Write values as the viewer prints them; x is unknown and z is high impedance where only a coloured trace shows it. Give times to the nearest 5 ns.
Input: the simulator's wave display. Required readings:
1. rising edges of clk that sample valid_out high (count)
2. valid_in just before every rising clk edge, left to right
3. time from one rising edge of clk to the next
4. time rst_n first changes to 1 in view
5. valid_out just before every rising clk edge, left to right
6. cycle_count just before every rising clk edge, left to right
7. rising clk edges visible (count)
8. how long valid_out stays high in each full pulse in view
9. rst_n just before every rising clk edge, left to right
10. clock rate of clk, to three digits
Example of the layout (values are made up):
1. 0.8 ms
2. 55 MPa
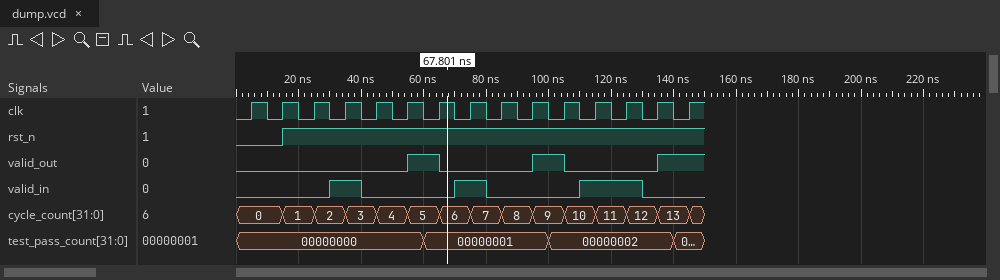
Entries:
1. 3
2. 0 0 0 1 0 0 0 1 0 0 0 1 1 0 0
3. 10 ns
4. 15 ns
5. 0 0 0 0 0 0 1 0 0 0 1 0 0 0 1
6. 0, 0, 1, 2, 3, 4, 5, 6, 7, 8, 9, 10, 11, 12, 13
7. 15
8. 10 ns, 10 ns
9. 0 0 1 1 1 1 1 1 1 1 1 1 1 1 1
10. 100 MHz
